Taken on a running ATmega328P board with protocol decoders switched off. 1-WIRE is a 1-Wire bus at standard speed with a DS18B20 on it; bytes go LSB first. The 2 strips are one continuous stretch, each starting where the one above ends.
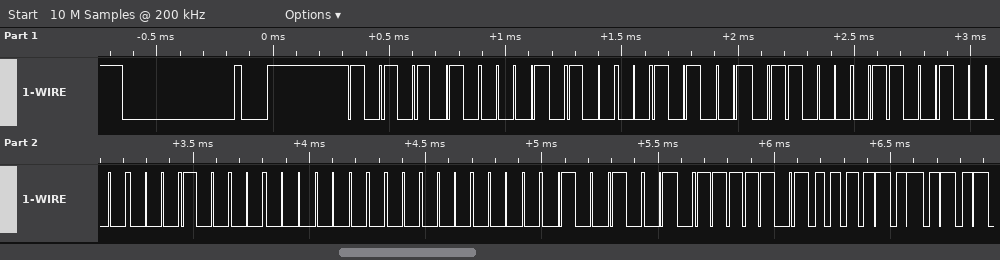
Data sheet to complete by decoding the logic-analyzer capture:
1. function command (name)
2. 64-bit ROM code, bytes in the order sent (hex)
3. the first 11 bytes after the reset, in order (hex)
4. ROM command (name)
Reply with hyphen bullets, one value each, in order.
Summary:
- Read Scratchpad
- 28 94 86 09 08 00 00 92
- 55 28 94 86 09 08 00 00 92 BE 50
- Match ROM
